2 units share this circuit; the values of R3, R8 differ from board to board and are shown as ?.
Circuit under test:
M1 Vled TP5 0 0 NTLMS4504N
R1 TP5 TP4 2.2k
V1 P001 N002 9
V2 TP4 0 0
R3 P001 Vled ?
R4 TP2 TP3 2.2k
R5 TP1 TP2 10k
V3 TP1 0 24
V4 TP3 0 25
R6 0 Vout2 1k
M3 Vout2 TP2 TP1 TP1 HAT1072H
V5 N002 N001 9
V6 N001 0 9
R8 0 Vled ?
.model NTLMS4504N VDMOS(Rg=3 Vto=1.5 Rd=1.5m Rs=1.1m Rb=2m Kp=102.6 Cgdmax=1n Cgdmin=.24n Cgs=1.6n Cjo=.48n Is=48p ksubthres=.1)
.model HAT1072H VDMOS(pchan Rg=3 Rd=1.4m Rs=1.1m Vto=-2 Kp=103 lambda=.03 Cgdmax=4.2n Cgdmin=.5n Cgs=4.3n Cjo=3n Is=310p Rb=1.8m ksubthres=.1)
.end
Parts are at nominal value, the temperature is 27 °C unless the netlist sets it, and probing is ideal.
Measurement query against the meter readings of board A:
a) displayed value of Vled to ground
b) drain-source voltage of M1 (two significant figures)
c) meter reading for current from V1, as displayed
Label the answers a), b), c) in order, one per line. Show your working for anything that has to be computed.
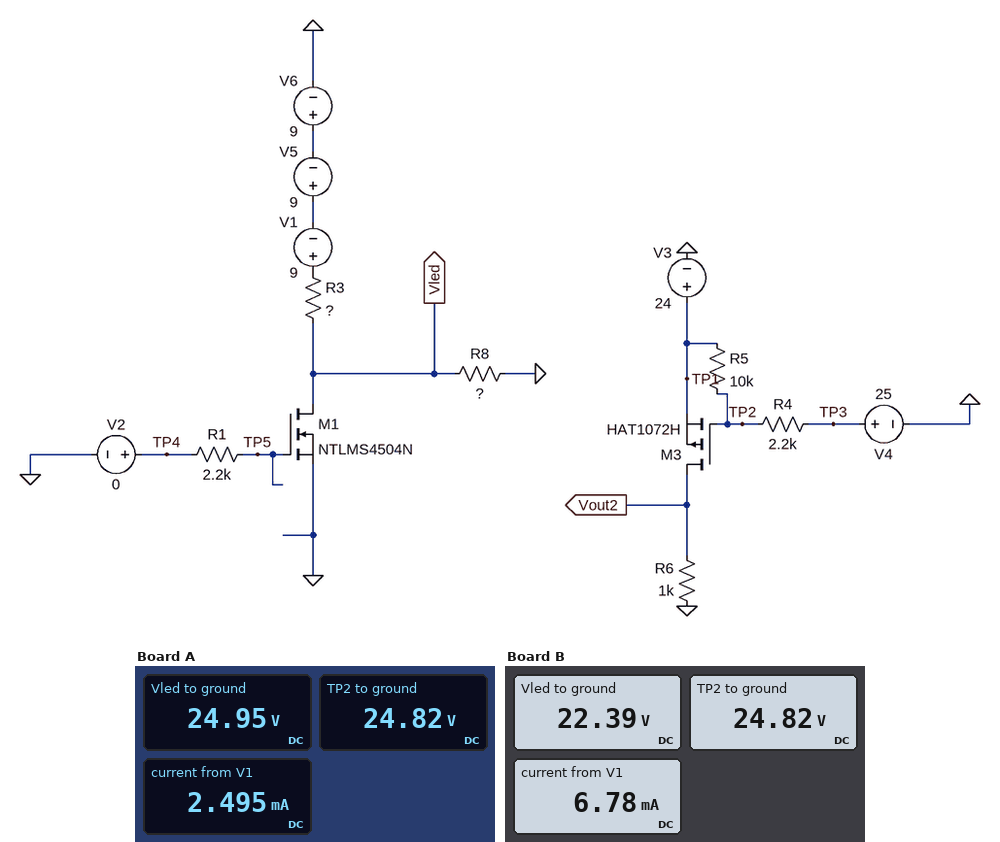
a) 24.95 V
b) 24.95 V = 25 V
c) 2.495 mA
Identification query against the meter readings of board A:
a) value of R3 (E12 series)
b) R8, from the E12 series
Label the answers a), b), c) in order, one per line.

a) 820 Ω
b) 10 kΩ
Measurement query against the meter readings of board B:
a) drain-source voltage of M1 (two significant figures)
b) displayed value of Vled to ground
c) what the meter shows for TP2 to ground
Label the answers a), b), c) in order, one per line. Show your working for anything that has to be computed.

a) 22.39 V = 22 V
b) 22.39 V
c) 24.82 V
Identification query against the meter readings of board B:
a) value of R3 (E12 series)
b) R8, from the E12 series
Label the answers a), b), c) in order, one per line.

a) 680 Ω
b) 3.3 kΩ
